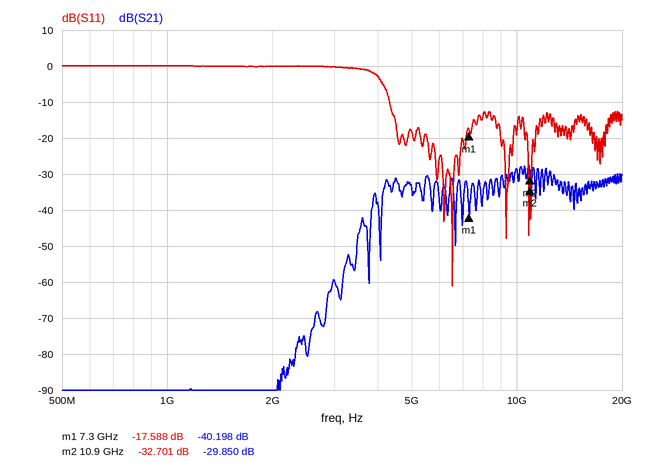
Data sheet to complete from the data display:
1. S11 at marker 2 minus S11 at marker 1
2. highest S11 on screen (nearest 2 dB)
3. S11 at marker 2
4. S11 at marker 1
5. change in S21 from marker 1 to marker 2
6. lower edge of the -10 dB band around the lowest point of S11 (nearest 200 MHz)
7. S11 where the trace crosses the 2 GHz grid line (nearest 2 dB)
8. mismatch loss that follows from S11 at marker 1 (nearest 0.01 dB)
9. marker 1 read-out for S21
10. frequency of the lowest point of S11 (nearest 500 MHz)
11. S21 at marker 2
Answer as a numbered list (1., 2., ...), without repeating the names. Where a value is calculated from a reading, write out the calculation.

1. -32.701 − (-17.588) = -15.113 dB
2. 0 dB
3. -32.701 dB
4. -17.588 dB
5. -29.85 − (-40.198) = 10.348 dB
6. 4.4 GHz
7. 0 dB
8. −10 log10(1 − 10^(-17.588/10)) ≈ 0.08 dB
9. -40.198 dB
10. 6.5 GHz
11. -29.850 dB
